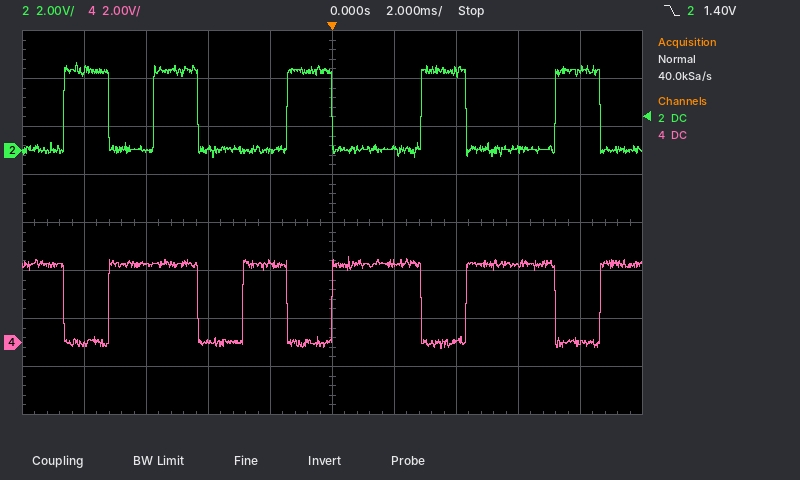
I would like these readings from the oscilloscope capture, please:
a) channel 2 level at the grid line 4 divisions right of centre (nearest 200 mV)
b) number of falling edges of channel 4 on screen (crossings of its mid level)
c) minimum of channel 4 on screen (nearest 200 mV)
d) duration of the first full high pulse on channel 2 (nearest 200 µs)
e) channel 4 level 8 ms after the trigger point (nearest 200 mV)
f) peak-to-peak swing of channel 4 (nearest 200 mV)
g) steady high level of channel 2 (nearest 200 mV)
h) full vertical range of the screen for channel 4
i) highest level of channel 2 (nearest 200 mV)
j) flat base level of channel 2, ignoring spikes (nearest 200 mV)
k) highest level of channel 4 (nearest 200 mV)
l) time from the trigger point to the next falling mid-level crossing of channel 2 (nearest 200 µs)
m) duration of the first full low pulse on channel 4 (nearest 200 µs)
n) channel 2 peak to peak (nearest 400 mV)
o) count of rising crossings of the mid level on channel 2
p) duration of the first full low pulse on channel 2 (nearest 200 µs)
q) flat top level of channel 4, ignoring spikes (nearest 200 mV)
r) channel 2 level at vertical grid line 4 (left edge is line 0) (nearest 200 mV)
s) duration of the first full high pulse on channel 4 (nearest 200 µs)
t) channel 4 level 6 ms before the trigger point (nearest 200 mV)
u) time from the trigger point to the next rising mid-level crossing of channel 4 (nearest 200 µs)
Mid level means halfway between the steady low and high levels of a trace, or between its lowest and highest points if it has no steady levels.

3.4 V
5
-200 mV
1.4 ms
0.0 V
3.8 V
3.4 V
16 V
3.6 V
0.0 V
3.6 V
4.4 ms
1.4 ms
4.0 V
5
1.4 ms
3.2 V
0.0 V
2.8 ms
3.2 V
4.4 ms
